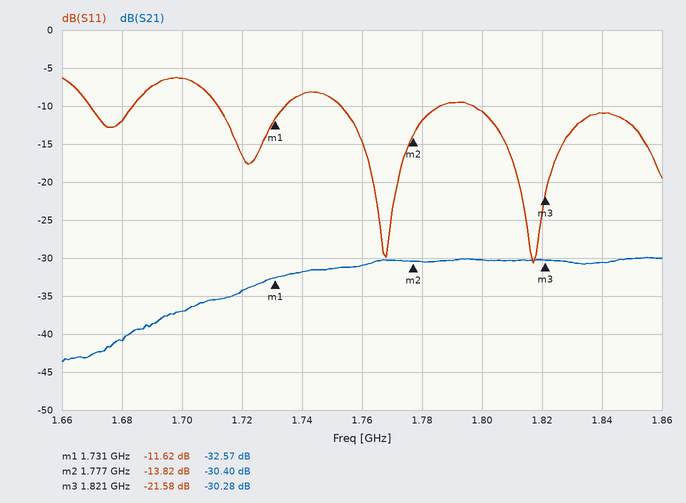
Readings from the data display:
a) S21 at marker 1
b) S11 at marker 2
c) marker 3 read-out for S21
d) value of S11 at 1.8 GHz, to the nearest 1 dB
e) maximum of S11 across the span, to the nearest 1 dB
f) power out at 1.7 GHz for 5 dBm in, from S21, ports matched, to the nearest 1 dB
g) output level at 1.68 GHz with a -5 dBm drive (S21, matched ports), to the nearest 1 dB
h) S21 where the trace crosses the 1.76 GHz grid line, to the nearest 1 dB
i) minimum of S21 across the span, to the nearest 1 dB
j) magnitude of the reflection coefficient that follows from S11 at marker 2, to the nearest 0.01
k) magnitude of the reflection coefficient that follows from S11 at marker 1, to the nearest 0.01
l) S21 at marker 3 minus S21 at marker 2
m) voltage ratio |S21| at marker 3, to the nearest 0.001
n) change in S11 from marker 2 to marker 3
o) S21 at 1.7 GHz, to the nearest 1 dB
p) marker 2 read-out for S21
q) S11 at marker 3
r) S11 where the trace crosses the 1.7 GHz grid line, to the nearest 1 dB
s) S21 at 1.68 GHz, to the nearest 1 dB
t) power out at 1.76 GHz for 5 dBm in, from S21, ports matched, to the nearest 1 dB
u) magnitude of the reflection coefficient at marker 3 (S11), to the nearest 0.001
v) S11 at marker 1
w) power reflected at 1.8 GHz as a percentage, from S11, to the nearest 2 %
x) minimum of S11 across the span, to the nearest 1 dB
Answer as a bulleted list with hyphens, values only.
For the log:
- -32.57 dB
- -13.82 dB
- -30.28 dB
- -11 dB
- -6 dB
- -32 dBm
- -46 dBm
- -31 dB
- -44 dB
- 0.20
- 0.26
- 0.12 dB
- 0.031
- -7.76 dB
- -37 dB
- -30.40 dB
- -21.58 dB
- -6 dB
- -41 dB
- -26 dBm
- 0.083
- -11.62 dB
- 8 %
- -31 dB
